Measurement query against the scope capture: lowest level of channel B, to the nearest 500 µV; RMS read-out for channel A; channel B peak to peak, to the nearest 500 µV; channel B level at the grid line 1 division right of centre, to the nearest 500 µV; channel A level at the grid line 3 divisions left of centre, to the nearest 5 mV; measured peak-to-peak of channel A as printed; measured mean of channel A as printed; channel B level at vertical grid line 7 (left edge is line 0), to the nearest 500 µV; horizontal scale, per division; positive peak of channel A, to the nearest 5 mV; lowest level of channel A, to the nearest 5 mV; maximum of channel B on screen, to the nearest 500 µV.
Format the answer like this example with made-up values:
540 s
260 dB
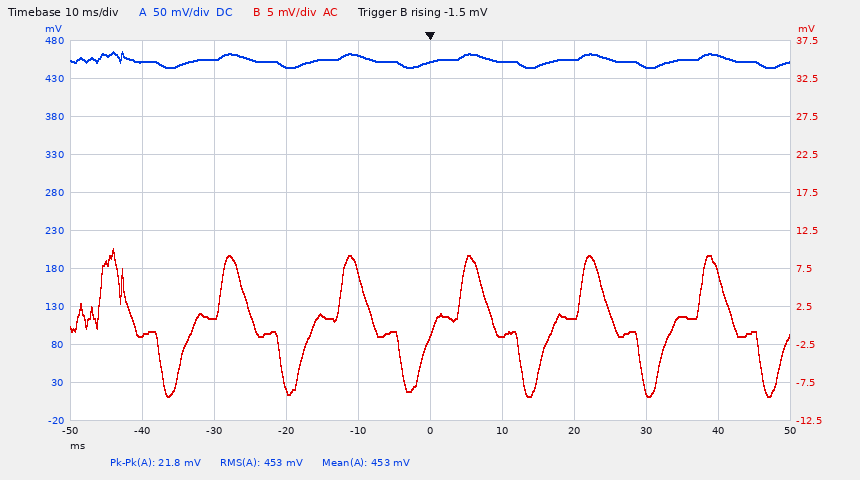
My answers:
-9.5 mV
453 mV
19.5 mV
-1.5 mV
455 mV
21.8 mV
453 mV
1.0 mV
10 ms
465 mV
445 mV
10.0 mV
